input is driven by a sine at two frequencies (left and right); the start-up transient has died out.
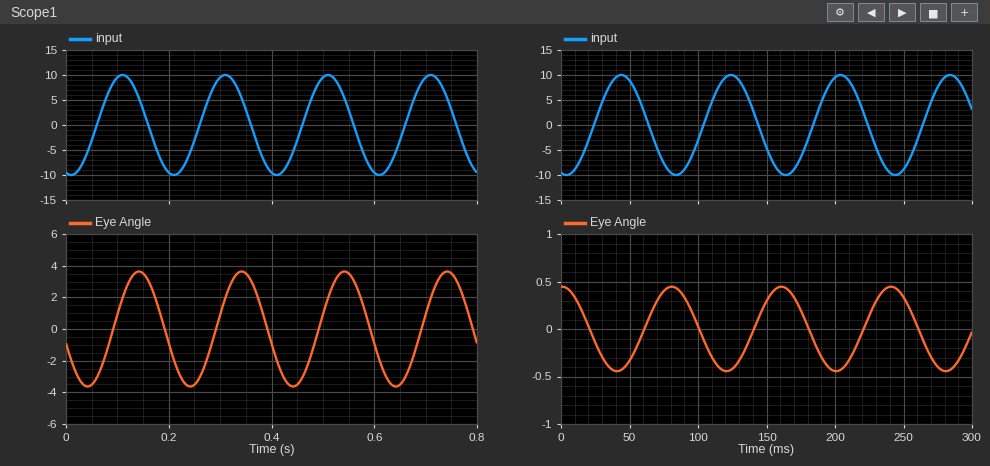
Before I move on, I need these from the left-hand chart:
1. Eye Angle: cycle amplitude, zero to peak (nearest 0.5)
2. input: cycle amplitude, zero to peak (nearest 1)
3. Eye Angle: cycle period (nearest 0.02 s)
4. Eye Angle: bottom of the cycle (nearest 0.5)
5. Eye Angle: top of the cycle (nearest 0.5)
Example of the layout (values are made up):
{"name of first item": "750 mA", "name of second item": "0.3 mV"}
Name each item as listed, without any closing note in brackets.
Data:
{"Eye Angle: cycle amplitude, zero to peak": "3.5", "input: cycle amplitude, zero to peak": "10", "Eye Angle: cycle period": "0.20 s", "Eye Angle: bottom of the cycle": "-3.5", "Eye Angle: top of the cycle": "3.5"}
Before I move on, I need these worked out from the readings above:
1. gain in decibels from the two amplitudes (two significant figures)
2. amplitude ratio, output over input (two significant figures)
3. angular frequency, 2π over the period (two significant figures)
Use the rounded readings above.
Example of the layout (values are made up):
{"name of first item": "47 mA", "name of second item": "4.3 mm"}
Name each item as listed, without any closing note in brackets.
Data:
{"gain in decibels from the two amplitudes": "-9.1 dB", "amplitude ratio, output over input": "0.35", "angular frequency, 2π over the period": "31 rad/s"}
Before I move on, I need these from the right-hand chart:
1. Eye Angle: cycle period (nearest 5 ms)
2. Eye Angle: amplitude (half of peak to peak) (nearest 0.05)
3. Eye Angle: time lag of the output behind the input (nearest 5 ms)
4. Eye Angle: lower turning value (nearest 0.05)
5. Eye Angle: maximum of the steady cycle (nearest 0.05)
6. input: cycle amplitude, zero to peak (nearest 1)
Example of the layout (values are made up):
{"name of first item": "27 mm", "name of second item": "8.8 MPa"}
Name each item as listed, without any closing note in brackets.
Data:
{"Eye Angle: cycle period": "80 ms", "Eye Angle: amplitude (half of peak to peak)": "0.45", "Eye Angle: time lag of the output behind the input": "35 ms", "Eye Angle: lower turning value": "-0.45", "Eye Angle: maximum of the steady cycle": "0.45", "input: cycle amplitude, zero to peak": "10"}
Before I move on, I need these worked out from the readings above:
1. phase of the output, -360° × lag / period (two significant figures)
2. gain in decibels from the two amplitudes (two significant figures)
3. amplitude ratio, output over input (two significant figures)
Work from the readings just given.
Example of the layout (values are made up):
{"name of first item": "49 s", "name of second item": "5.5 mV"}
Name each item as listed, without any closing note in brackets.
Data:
{"phase of the output, -360° × lag / period": "-160°", "gain in decibels from the two amplitudes": "-27 dB", "amplitude ratio, output over input": "0.045"}
